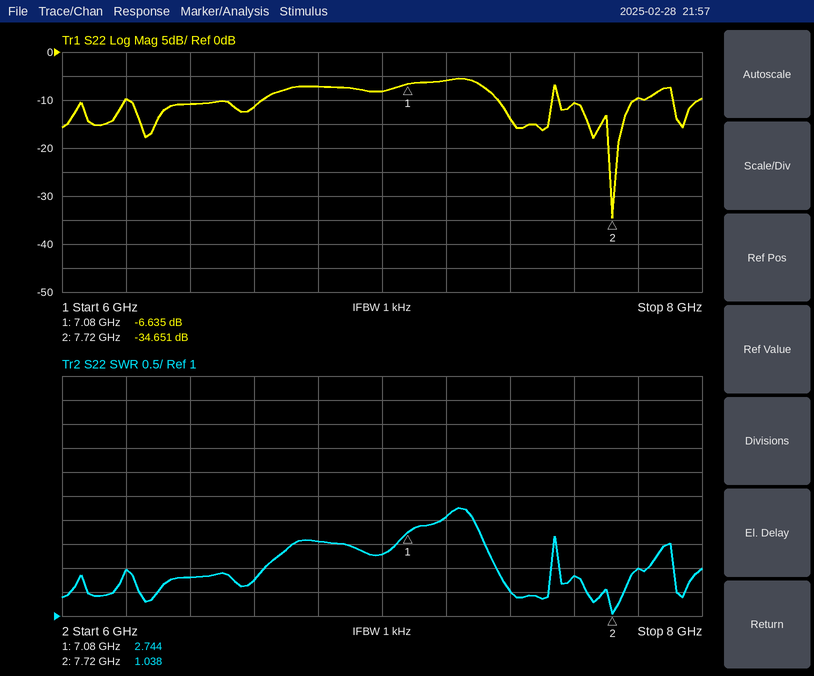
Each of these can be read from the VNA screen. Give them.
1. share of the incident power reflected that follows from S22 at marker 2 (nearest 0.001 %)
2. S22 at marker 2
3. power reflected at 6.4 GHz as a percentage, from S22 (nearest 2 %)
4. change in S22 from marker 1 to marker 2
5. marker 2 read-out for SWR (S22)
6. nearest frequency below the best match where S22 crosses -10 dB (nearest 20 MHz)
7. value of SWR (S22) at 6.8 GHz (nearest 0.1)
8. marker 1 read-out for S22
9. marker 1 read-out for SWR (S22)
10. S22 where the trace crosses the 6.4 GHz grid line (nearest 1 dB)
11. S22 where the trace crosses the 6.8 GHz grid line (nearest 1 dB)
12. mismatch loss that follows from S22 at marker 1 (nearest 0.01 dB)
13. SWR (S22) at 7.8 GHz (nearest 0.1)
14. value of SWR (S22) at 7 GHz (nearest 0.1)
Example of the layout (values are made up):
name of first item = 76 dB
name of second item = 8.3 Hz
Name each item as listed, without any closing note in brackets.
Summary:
share of the incident power reflected that follows from S22 at marker 2 = 0.034 %
S22 at marker 2 = -34.651 dB
power reflected at 6.4 GHz as a percentage, from S22 = 8 %
change in S22 from marker 1 to marker 2 = -28.016 dB
marker 2 read-out for SWR = 1.038
nearest frequency below the best match where S22 crosses -10 dB = 7.56 GHz
value of SWR (S22) at 6.8 GHz = 2.6
marker 1 read-out for S22 = -6.635 dB
marker 1 read-out for SWR = 2.744
S22 where the trace crosses the 6.4 GHz grid line = -11 dB
S22 where the trace crosses the 6.8 GHz grid line = -7 dB
mismatch loss that follows from S22 at marker 1 = 1.06 dB
SWR (S22) at 7.8 GHz = 2.0
value of SWR (S22) at 7 GHz = 2.3
